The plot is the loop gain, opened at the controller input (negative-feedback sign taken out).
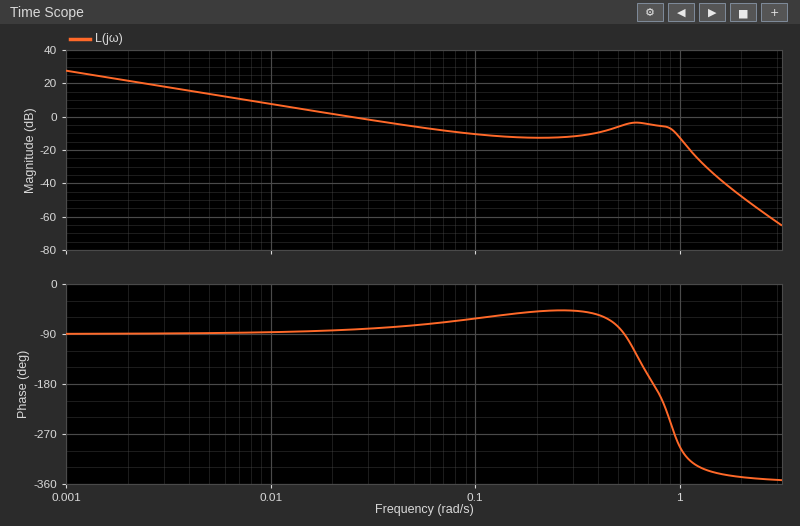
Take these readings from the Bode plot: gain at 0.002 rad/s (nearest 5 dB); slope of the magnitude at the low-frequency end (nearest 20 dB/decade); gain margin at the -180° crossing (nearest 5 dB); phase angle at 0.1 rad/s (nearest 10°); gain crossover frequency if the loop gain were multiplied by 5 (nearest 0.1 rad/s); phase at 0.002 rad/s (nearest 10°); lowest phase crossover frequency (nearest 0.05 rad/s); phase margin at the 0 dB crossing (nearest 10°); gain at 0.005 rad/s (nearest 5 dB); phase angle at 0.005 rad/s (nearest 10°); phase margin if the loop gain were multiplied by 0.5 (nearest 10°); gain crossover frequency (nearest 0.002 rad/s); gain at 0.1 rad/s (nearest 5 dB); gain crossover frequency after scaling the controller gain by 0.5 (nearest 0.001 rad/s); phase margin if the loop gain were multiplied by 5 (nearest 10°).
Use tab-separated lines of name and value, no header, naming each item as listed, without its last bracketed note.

gain at 0.002 rad/s	20 dB
slope of the magnitude at the low-frequency end	-20 dB/decade
gain margin at the -180° crossing	5 dB
phase angle at 0.1 rad/s	-60°
gain crossover frequency if the loop gain were multiplied by 5	1.0 rad/s
phase at 0.002 rad/s	-90°
lowest phase crossover frequency	0.75 rad/s
phase margin at the 0 dB crossing	100°
gain at 0.005 rad/s	15 dB
phase angle at 0.005 rad/s	-90°
phase margin if the loop gain were multiplied by 0.5	90°
gain crossover frequency	0.024 rad/s
gain at 0.1 rad/s	-10 dB
gain crossover frequency after scaling the controller gain by 0.5	0.012 rad/s
phase margin if the loop gain were multiplied by 5	-120°
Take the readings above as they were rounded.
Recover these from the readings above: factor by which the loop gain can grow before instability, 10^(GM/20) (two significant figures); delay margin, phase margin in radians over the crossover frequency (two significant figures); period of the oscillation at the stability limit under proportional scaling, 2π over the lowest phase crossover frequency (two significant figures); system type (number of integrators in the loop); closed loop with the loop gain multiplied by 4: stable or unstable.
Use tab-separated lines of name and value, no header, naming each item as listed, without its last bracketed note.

factor by which the loop gain can grow before instability, 10^(GM/20)	1.8
delay margin, phase margin in radians over the crossover frequency	73 s
period of the oscillation at the stability limit under proportional scaling, 2π over the lowest phase crossover frequency	8.4 s
system type	1
closed loop with the loop gain multiplied by 4: stable or unstable	unstable
